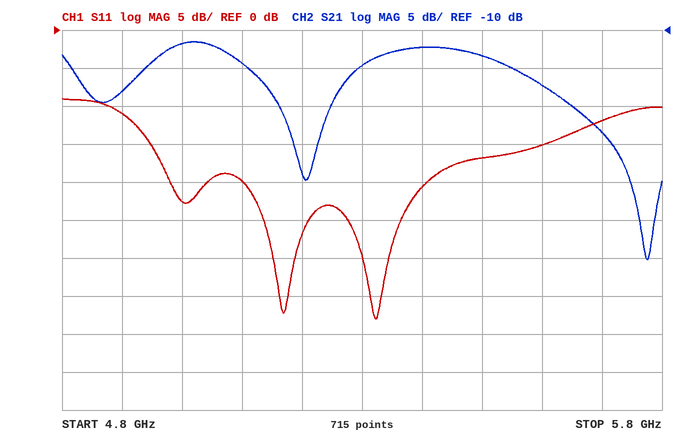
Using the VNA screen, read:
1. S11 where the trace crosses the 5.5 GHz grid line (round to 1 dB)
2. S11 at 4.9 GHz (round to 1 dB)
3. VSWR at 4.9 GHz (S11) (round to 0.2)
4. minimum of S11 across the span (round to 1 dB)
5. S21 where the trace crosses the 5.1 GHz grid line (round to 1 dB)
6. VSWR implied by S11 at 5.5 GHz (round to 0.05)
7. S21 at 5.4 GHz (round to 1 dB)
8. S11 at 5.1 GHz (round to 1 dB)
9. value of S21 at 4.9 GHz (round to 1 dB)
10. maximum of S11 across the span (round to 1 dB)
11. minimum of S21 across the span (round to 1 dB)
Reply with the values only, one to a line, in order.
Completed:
-17 dB
-11 dB
1.8
-38 dB
-14 dB
1.35
-12 dB
-20 dB
-18 dB
-9 dB
-40 dB
